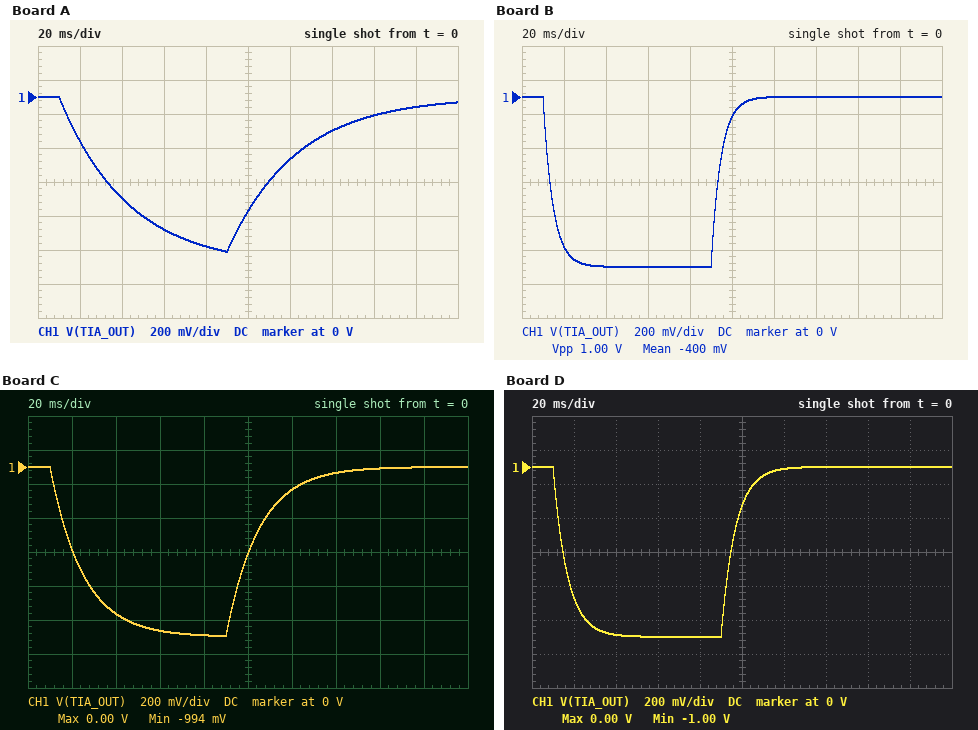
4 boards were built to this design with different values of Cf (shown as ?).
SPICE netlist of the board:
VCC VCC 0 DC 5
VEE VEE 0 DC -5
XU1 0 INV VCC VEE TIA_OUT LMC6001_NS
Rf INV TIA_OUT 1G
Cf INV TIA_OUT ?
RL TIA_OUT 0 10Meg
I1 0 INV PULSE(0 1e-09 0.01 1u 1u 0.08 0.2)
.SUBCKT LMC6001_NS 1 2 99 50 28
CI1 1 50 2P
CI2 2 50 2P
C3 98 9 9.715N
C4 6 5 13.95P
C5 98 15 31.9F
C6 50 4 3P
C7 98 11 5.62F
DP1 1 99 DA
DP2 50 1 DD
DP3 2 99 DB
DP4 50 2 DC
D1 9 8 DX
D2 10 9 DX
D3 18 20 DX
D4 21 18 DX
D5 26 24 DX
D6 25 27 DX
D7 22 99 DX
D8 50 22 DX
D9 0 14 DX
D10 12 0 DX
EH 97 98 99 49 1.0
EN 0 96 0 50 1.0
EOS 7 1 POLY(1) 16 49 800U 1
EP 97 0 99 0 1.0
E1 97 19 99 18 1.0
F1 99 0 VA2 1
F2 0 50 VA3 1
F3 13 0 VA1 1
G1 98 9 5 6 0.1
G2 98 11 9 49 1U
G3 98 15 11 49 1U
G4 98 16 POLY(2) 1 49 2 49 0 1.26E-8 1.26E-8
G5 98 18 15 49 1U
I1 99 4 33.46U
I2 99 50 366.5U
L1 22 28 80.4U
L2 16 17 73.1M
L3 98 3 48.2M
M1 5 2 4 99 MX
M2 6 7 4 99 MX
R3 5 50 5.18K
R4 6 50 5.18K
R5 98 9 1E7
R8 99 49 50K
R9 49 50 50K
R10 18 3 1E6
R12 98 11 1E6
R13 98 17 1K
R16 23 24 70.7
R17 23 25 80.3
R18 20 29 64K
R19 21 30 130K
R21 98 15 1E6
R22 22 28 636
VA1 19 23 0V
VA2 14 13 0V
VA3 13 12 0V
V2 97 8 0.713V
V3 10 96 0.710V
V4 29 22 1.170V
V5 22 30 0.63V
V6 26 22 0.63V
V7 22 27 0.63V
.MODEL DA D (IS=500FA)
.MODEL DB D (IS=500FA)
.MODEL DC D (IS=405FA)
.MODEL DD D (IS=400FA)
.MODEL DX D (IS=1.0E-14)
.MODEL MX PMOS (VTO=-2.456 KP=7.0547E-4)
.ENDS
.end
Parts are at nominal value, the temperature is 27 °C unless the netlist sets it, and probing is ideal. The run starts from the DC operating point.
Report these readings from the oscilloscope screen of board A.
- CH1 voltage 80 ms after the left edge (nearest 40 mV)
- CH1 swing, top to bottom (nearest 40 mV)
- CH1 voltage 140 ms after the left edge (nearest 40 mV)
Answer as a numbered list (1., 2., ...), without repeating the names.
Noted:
1. -880 mV
2. 920 mV
3. -200 mV
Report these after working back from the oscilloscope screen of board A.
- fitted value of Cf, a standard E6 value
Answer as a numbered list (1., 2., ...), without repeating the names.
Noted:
1. 33 pF
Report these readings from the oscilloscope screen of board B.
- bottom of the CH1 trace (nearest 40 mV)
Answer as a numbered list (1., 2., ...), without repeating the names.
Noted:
1. -1.00 V
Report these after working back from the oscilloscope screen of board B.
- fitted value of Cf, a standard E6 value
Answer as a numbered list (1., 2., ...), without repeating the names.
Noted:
1. 4.7 pF
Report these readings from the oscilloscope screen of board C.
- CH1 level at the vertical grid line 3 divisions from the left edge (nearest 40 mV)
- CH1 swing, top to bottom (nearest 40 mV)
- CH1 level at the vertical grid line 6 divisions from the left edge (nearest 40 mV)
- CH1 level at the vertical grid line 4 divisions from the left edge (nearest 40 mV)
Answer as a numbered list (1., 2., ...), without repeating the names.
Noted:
1. -960 mV
2. 1.00 V
3. -120 mV
4. -1.00 V
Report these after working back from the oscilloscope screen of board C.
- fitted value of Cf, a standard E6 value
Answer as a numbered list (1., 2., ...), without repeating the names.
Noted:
1. 15 pF
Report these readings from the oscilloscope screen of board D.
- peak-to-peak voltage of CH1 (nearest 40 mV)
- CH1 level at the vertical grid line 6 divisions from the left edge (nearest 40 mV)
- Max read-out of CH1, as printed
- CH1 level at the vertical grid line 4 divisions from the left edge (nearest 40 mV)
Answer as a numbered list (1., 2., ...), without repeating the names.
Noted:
1. 1.00 V
2. 0 V
3. 0.00 V
4. -1.00 V
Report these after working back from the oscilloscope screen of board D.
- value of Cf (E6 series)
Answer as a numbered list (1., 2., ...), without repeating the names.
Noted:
1. 6.8 pF
